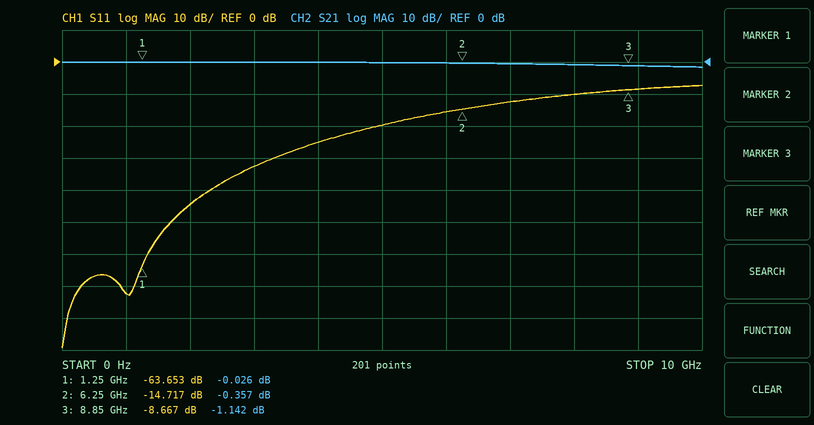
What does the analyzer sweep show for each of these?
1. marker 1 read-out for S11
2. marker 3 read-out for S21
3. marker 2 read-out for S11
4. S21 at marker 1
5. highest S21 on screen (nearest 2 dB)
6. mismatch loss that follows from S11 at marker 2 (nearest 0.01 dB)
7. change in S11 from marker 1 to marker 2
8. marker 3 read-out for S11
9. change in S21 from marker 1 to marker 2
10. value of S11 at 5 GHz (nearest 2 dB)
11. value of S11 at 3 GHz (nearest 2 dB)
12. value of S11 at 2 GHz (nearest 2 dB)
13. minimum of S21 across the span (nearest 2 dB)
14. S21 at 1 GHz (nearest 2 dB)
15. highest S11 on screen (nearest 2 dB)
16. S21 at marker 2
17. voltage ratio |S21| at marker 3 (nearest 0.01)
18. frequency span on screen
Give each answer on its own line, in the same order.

-63.653 dB
-1.142 dB
-14.717 dB
-0.026 dB
0 dB
0.15 dB
48.936 dB
-8.667 dB
-0.331 dB
-20 dB
-32 dB
-44 dB
-2 dB
0 dB
-8 dB
-0.357 dB
0.88
10 GHz
